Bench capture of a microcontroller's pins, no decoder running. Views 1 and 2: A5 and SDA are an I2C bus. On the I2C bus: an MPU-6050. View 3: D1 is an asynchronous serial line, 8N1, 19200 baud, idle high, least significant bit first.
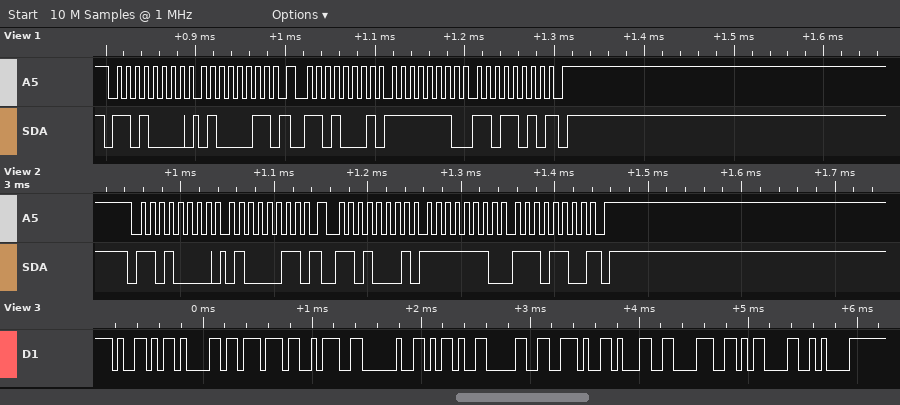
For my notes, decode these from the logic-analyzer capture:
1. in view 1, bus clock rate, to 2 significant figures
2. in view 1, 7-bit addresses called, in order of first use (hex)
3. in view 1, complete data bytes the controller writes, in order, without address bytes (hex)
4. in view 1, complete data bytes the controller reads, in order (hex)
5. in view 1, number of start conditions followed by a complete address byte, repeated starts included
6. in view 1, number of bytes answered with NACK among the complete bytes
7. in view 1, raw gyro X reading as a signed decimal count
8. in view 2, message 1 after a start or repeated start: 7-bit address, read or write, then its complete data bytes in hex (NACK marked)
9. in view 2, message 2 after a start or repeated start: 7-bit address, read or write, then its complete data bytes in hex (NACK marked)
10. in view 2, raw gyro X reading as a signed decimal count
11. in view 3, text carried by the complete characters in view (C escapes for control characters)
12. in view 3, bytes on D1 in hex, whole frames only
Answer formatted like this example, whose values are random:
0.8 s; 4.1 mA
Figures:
100 kHz; 0x68; 43; FE DA; 2; 1; -294; 0x68 write: 43; 0x68 read: FE EC NACK; -276; "Yaw: -0.18\r\n"; 59 61 77 3A 20 2D 30 2E 31 38 0D 0A
